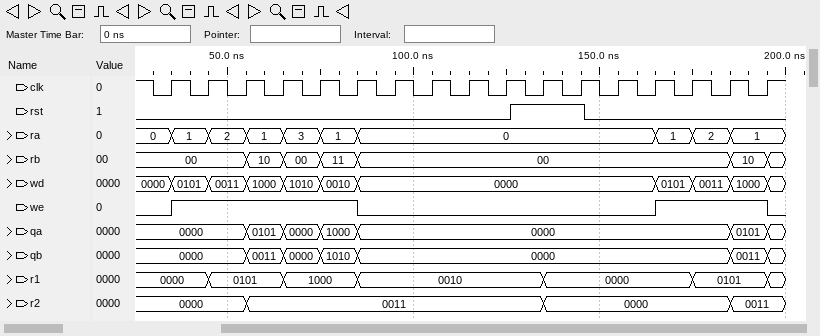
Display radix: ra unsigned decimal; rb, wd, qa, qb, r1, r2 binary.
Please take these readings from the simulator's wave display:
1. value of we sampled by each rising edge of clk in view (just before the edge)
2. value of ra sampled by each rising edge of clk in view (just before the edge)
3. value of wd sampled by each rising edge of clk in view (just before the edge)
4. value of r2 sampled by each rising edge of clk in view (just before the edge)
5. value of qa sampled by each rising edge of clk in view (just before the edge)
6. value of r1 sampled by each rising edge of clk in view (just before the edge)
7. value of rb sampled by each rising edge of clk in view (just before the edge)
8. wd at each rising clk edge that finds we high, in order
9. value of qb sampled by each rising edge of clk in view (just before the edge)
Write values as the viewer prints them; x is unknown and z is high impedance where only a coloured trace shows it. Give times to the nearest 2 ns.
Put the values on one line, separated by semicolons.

0 1 1 1 1 1 0 0 0 0 0 0 0 0 1 1 1; 0, 1, 2, 1, 3, 1, 0, 0, 0, 0, 0, 0, 0, 0, 1, 2, 1; 0000, 0101, 0011, 1000, 1010, 0010, 0000, 0000, 0000, 0000, 0000, 0000, 0000, 0000, 0101, 0011, 1000; 0000, 0000, 0000, 0011, 0011, 0011, 0011, 0011, 0011, 0011, 0011, 0000, 0000, 0000, 0000, 0000, 0011; 0000, 0000, 0000, 0101, 0000, 1000, 0000, 0000, 0000, 0000, 0000, 0000, 0000, 0000, 0000, 0000, 0101; 0000, 0000, 0101, 0101, 1000, 1000, 0010, 0010, 0010, 0010, 0010, 0000, 0000, 0000, 0000, 0101, 0101; 00, 00, 00, 10, 00, 11, 00, 00, 00, 00, 00, 00, 00, 00, 00, 00, 10; 0101, 0011, 1000, 1010, 0010, 0101, 0011, 1000; 0000, 0000, 0000, 0011, 0000, 1010, 0000, 0000, 0000, 0000, 0000, 0000, 0000, 0000, 0000, 0000, 0011
